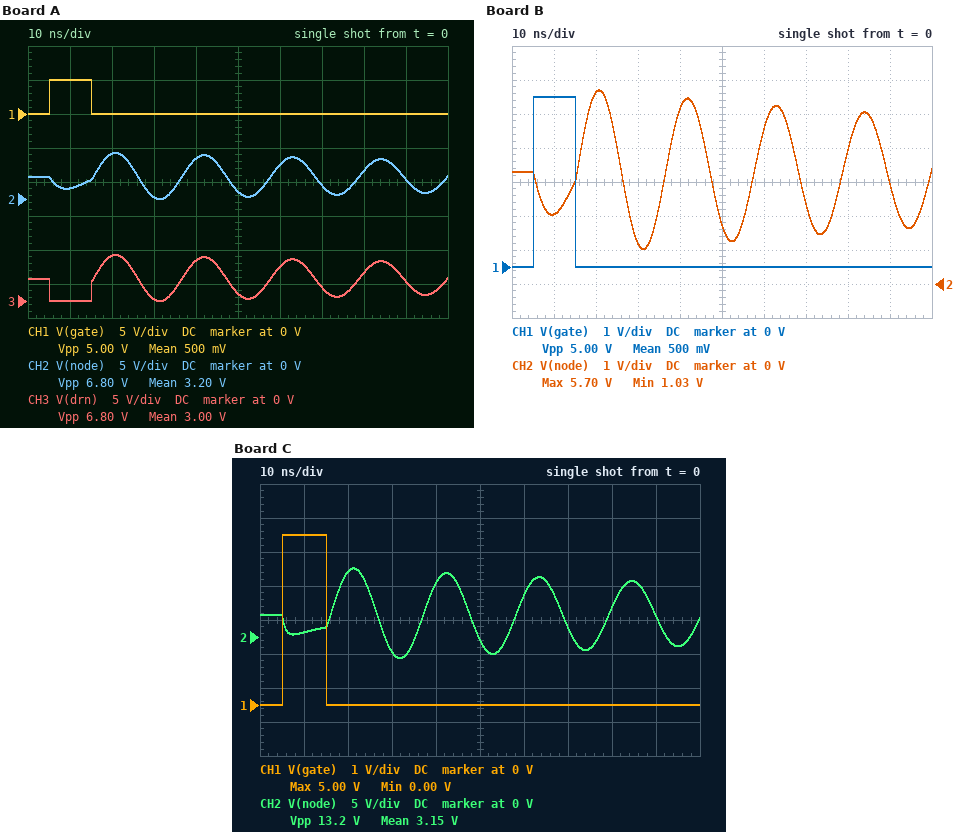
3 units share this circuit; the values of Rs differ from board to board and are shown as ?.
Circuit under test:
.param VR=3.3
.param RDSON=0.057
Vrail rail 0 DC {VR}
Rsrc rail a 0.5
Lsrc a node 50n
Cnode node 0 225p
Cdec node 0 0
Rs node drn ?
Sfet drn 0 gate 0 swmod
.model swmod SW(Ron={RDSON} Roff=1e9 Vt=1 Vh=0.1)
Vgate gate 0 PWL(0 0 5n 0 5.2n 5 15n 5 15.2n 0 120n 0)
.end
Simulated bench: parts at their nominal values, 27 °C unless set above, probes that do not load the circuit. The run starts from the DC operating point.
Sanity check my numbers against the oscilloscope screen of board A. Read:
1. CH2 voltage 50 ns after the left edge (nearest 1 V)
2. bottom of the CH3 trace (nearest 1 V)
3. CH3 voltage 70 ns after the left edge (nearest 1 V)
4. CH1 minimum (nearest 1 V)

1 V
0 V
2 V
0 V
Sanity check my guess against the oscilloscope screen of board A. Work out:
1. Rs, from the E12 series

15 Ω
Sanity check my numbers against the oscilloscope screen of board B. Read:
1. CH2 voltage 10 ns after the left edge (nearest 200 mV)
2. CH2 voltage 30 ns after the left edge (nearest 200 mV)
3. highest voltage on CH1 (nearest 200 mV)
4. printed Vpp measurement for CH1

2.0 V
1.2 V
5.0 V
5.00 V
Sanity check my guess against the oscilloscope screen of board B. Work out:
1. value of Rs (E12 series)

27 Ω
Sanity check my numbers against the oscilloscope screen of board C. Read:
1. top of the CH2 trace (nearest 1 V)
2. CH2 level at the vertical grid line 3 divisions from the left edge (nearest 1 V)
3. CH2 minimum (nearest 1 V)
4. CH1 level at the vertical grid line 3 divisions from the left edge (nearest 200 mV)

10 V
-2 V
-3 V
0 V
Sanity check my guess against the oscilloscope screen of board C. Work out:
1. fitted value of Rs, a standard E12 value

3.3 Ω
